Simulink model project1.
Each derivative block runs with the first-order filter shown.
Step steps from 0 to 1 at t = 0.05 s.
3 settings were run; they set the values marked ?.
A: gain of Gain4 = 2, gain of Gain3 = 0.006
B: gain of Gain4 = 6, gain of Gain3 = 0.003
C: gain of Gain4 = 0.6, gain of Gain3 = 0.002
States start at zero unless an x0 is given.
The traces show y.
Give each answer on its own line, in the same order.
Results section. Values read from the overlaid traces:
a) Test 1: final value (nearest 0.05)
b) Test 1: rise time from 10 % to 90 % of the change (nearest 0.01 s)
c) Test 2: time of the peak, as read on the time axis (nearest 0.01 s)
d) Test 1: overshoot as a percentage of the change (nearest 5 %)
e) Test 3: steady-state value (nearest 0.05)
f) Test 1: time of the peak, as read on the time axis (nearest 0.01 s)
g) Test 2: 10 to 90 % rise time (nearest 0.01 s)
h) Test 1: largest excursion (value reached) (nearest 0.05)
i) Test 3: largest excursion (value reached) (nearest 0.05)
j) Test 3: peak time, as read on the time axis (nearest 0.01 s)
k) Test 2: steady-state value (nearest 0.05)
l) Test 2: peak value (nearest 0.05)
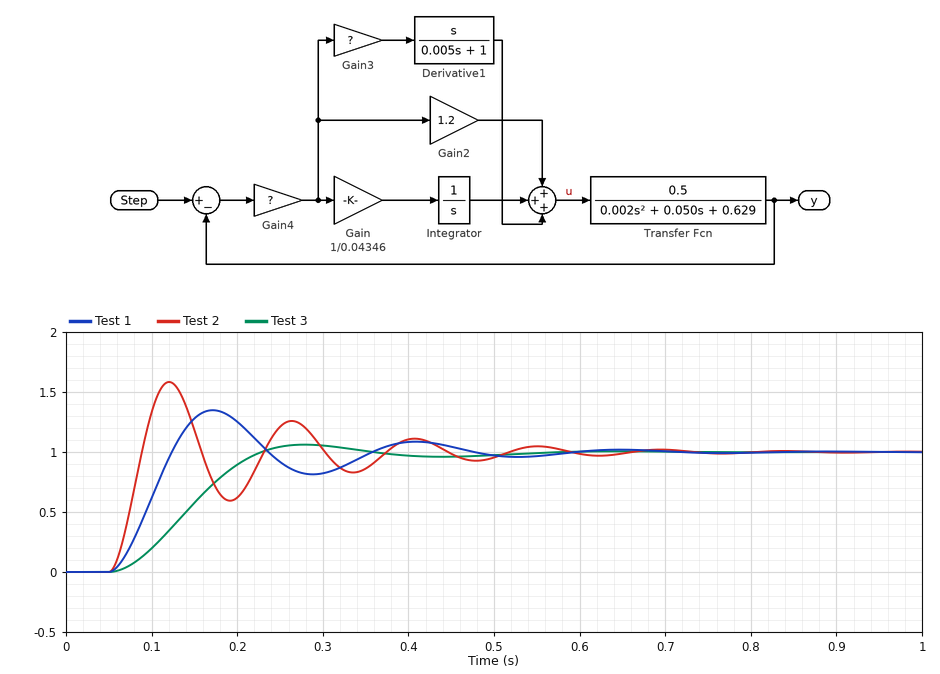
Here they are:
1.00
0.05 s
0.12 s
35 %
1.00
0.17 s
0.03 s
1.35
1.05
0.28 s
1.00
1.60
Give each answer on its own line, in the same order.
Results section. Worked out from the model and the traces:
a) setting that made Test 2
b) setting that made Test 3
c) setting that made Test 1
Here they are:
B
C
A
